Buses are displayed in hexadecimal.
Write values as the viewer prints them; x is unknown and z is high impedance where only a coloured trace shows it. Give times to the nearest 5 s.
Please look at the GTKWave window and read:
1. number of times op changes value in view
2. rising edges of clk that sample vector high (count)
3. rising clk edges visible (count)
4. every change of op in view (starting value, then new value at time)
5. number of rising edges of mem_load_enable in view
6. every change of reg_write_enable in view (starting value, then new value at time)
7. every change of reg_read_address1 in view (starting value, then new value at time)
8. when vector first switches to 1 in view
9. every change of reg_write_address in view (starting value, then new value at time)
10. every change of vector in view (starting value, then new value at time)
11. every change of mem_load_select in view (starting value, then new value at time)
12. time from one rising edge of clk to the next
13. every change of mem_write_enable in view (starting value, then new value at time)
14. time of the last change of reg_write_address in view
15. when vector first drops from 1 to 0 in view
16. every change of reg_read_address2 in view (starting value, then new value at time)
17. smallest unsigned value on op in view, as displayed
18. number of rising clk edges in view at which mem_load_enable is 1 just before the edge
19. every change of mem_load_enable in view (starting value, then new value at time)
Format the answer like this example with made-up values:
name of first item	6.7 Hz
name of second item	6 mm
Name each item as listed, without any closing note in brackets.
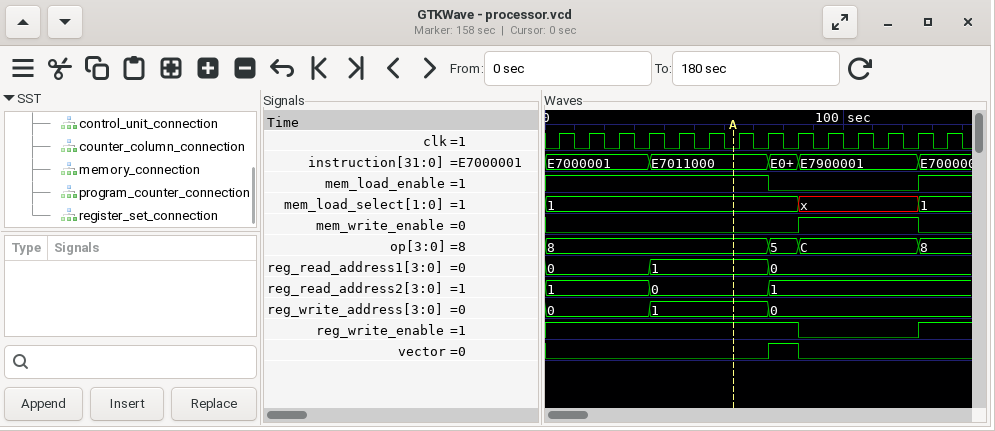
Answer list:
number of times op changes value in view	3
rising edges of clk that sample vector high	1
rising clk edges visible	14
every change of op in view	8, 5 at 75 s, C at 85 s, 8 at 125 s
number of rising edges of mem_load_enable in view	1
every change of reg_write_enable in view	1, 0 at 85 s, 1 at 125 s
every change of reg_read_address1 in view	0, 1 at 35 s, 0 at 75 s
when vector first switches to 1 in view	75 s
every change of reg_write_address in view	0, 1 at 35 s, 0 at 75 s
every change of vector in view	0, 1 at 75 s, 0 at 85 s
every change of mem_load_select in view	1, x at 85 s, 1 at 125 s
time from one rising edge of clk to the next	10 s
every change of mem_write_enable in view	0, 1 at 85 s, 0 at 125 s
time of the last change of reg_write_address in view	75 s
when vector first drops from 1 to 0 in view	85 s
every change of reg_read_address2 in view	1, 0 at 35 s, 1 at 75 s
smallest unsigned value on op in view, as displayed	5
number of rising clk edges in view at which mem_load_enable is 1 just before the edge	9
every change of mem_load_enable in view	1, 0 at 75 s, 1 at 125 s
